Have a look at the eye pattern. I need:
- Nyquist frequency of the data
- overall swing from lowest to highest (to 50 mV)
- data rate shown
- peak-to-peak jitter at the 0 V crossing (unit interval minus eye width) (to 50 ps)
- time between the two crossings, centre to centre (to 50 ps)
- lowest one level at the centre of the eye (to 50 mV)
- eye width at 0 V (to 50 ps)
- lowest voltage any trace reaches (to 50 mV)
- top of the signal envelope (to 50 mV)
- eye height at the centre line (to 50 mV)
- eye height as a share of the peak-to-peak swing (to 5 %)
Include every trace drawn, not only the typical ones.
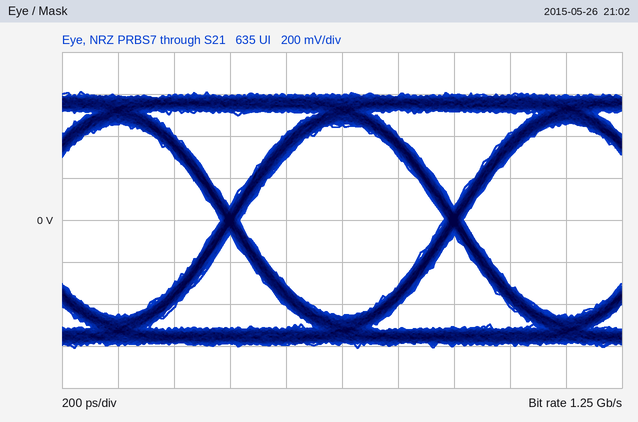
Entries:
625 MHz
1.20 V
1.25 Gb/s
50 ps
800 ps
450 mV
750 ps
-600 mV
600 mV
900 mV
75 %
